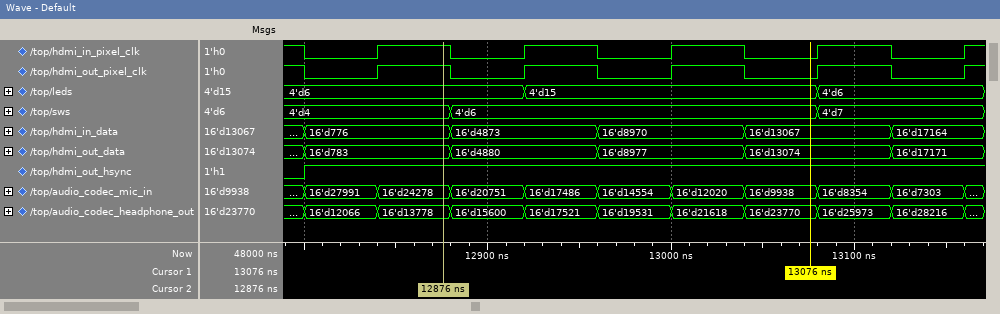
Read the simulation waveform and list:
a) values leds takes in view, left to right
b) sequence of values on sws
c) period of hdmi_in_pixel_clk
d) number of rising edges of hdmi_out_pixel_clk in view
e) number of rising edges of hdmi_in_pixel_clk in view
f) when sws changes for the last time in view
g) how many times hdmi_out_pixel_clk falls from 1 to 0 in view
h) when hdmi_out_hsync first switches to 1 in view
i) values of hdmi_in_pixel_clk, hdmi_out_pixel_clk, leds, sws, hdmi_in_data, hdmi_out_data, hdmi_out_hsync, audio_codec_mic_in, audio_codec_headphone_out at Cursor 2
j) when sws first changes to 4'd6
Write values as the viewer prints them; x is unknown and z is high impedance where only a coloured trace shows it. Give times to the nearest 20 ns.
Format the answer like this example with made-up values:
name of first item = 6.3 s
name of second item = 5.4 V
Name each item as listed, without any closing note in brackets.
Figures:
values leds takes in view, left to right = 4'd6, 4'd15, 4'd6
sequence of values on sws = 4'd4, 4'd6, 4'd7
period of hdmi_in_pixel_clk = 80 ns
number of rising edges of hdmi_out_pixel_clk in view = 5
number of rising edges of hdmi_in_pixel_clk in view = 5
when sws changes for the last time in view = 13080 ns
how many times hdmi_out_pixel_clk falls from 1 to 0 in view = 5
when hdmi_out_hsync first switches to 1 in view = 12800 ns
values of hdmi_in_pixel_clk, hdmi_out_pixel_clk, leds, sws, hdmi_in_data, hdmi_out_data, hdmi_out_hsync, audio_codec_mic_in, audio_codec_headphone_out at Cursor 2 = hdmi_in_pixel_clk=1, hdmi_out_pixel_clk=1, leds=4'd6, sws=4'd4, hdmi_in_data=16'd776, hdmi_out_data=16'd783, hdmi_out_hsync=1, audio_codec_mic_in=16'd24278, audio_codec_headphone_out=16'd13778
when sws first changes to 4'd6 = 12880 ns
